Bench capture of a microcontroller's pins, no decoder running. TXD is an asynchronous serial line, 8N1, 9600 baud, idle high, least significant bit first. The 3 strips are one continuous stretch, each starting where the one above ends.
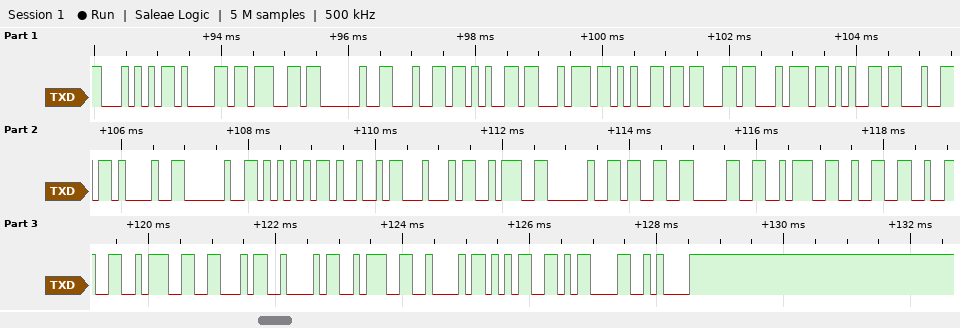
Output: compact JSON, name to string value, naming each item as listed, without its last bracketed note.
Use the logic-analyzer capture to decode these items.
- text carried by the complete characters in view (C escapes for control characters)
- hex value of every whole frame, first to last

{"text carried by the complete characters in view": "\"Tag detected! UID: 30:22:FB:B5\\r\\n\"", "hex value of every whole frame, first to last": "54 61 67 20 64 65 74 65 63 74 65 64 21 20 55 49 44 3A 20 33 30 3A 32 32 3A 46 42 3A 42 35 0D 0A"}
